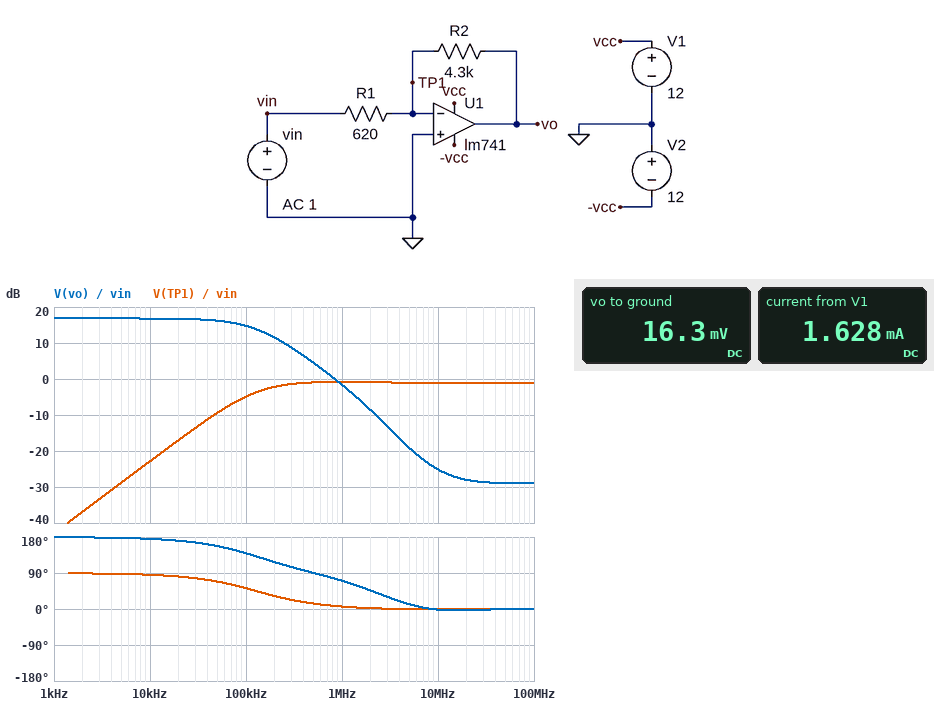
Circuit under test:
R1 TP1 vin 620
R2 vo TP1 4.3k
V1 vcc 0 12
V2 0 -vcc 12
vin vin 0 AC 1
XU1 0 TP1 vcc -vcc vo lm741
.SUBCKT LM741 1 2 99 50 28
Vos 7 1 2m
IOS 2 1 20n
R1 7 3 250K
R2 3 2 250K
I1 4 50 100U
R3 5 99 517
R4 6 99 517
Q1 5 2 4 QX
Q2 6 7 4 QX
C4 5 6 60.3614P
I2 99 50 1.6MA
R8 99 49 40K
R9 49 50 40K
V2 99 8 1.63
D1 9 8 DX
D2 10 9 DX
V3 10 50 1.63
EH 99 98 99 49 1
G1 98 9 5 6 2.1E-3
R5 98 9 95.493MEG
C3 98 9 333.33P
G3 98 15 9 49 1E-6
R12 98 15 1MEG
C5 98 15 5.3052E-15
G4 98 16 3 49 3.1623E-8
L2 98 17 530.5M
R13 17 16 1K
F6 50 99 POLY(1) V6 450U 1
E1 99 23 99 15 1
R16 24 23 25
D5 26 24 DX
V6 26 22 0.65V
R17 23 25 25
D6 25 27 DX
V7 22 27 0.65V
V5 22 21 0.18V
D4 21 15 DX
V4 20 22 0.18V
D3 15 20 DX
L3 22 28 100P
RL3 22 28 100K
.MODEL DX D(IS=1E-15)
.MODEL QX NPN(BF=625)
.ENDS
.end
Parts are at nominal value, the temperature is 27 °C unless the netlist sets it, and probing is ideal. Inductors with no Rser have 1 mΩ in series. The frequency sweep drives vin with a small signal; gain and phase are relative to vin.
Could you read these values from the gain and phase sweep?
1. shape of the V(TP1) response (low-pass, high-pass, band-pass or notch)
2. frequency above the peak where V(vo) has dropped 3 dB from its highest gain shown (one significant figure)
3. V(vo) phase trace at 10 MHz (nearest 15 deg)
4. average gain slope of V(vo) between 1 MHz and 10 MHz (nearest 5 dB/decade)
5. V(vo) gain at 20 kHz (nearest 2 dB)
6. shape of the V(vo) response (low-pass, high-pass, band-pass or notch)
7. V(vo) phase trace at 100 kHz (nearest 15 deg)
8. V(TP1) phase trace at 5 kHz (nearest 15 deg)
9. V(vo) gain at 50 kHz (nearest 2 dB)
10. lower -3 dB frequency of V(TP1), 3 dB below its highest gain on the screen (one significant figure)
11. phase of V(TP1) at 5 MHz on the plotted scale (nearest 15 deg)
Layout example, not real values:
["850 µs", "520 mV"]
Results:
["high-pass", "100 kHz", "0 deg", "-25 dB/decade", "16 dB", "low-pass", "135 deg", "90 deg", "16 dB", "100 kHz", "0 deg"]
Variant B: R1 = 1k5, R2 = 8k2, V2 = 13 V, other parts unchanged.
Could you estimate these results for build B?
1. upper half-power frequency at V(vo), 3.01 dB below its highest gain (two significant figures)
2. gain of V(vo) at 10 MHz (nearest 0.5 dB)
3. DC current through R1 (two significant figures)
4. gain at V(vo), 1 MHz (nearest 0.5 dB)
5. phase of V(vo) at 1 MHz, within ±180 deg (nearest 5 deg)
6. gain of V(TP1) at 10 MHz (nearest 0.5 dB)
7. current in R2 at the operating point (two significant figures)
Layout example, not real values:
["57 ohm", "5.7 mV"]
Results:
["160 kHz", "-28.5 dB", "1.3 µA", "-2.0 dB", "75 deg", "-1.5 dB", "1.4 µA"]
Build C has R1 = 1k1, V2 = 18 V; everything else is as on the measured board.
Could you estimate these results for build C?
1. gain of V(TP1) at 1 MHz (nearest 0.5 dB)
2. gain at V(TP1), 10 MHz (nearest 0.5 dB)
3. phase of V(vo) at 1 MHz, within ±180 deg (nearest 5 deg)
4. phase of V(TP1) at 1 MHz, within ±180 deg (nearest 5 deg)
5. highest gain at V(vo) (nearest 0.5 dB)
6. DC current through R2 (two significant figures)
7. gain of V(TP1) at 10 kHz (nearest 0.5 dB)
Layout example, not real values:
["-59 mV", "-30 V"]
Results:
["-1.5 dB", "-2.0 dB", "75 deg", "10 deg", "12.0 dB", "1.9 µA", "-28.0 dB"]
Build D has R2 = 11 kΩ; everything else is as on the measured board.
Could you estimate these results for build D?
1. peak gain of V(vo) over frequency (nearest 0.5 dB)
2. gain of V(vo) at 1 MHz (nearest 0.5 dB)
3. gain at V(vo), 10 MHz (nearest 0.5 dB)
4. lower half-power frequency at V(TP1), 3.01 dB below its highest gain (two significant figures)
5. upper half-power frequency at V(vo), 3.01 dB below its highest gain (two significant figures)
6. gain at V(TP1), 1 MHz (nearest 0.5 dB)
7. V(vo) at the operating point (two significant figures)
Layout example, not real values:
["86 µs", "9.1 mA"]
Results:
["25.0 dB", "-1.0 dB", "-28.5 dB", "53 kHz", "54 kHz", "-0.5 dB", "39 mV"]
